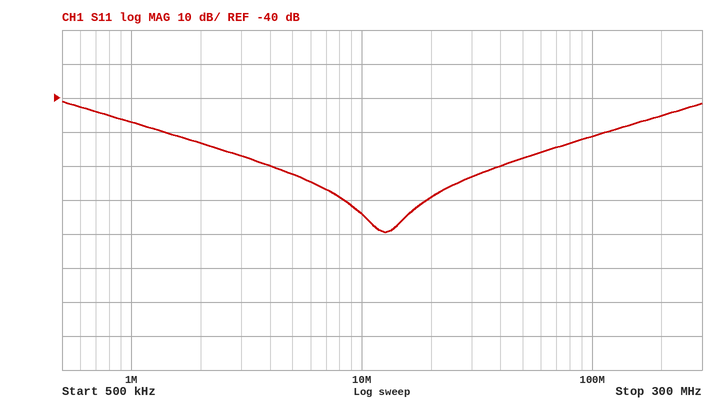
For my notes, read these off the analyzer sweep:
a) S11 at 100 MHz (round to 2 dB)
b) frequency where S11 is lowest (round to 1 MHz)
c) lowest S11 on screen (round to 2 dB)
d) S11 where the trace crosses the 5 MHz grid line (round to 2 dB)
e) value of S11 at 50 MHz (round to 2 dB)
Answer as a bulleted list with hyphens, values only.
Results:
- -52 dB
- 13 MHz
- -80 dB
- -62 dB
- -58 dB
